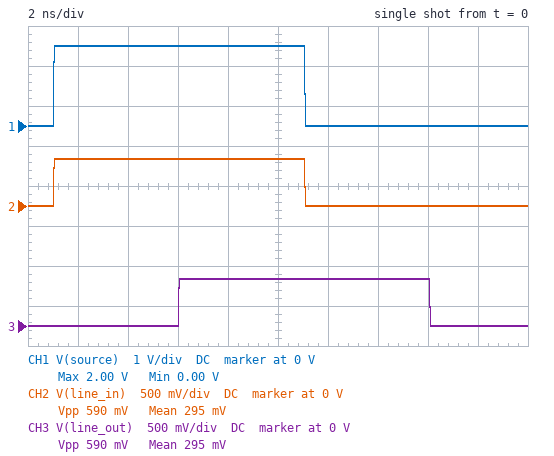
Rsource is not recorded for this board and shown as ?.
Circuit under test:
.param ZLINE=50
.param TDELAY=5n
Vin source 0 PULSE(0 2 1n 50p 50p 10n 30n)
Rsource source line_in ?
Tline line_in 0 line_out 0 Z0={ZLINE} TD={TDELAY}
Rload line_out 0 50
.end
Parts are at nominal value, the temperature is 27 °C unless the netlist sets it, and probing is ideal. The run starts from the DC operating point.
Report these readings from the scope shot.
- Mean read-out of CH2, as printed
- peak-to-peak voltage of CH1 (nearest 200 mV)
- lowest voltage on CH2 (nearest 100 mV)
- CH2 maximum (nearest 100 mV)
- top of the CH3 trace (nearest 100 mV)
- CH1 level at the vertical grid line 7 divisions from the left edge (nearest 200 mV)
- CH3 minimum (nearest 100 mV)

295 mV
2.0 V
0 V
600 mV
600 mV
0 V
0 V
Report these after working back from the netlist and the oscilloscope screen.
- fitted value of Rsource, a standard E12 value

120 Ω
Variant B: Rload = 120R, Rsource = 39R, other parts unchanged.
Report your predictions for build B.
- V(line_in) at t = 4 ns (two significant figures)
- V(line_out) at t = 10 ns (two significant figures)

1.1 V
1.6 V
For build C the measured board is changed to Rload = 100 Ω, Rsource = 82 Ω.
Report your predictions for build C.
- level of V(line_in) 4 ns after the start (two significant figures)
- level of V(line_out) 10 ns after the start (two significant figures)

760 mV
1.0 V
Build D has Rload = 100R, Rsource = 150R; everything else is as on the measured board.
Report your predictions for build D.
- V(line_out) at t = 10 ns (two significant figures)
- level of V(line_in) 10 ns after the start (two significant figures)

670 mV
500 mV
